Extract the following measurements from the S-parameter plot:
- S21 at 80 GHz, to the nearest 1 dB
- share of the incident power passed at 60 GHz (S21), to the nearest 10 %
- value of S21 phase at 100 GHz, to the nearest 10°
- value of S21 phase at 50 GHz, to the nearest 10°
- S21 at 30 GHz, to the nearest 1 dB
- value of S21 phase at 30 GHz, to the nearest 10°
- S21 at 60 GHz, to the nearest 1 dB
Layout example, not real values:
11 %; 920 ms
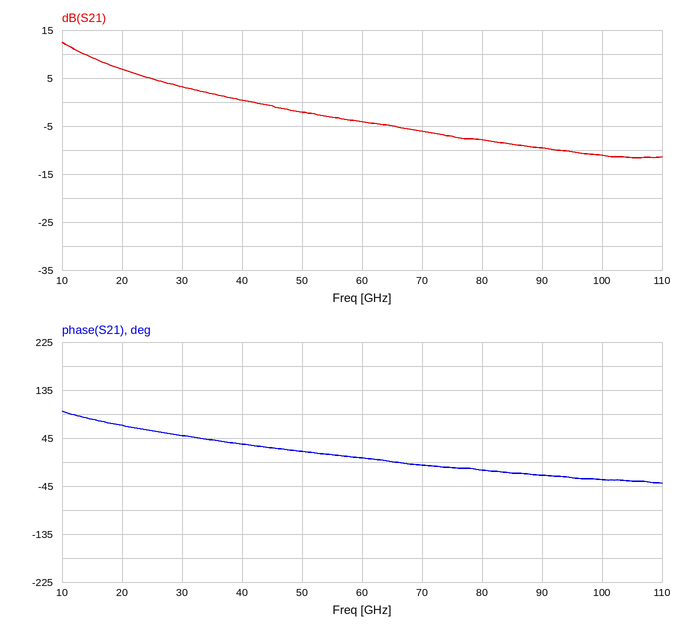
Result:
-8 dB; 40 %; -30°; 20°; 3 dB; 50°; -4 dB
